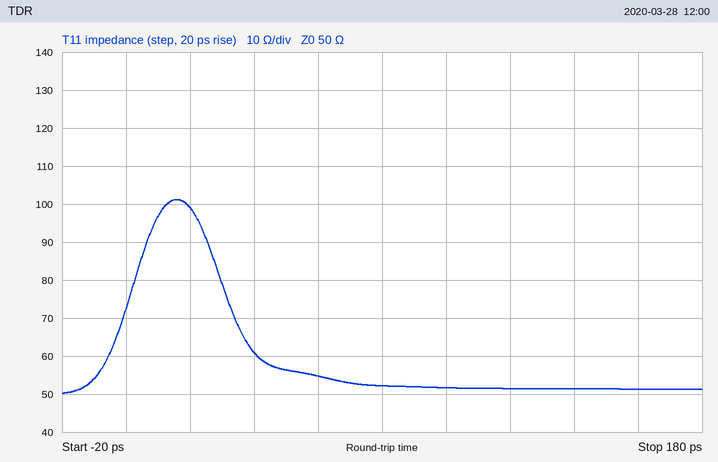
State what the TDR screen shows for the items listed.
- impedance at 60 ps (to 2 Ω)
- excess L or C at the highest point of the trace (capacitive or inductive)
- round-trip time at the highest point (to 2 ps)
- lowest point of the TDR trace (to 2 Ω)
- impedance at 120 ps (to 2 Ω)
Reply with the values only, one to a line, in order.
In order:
54 Ω
inductive
16 ps
50 Ω
52 Ω
